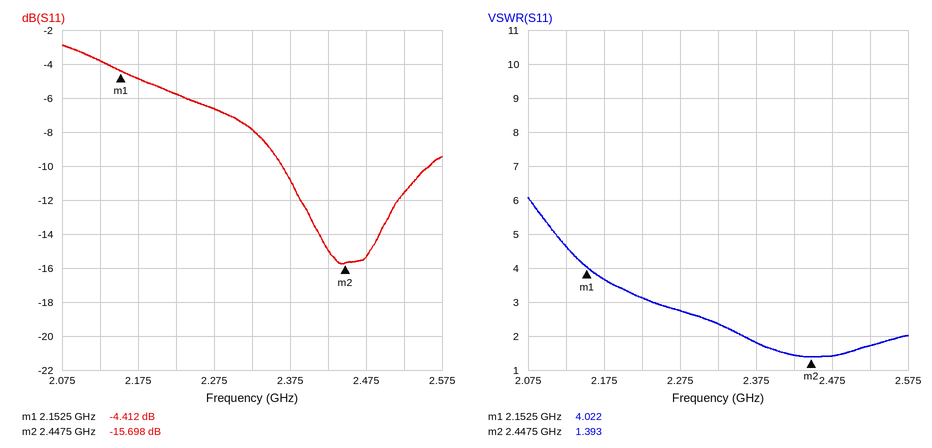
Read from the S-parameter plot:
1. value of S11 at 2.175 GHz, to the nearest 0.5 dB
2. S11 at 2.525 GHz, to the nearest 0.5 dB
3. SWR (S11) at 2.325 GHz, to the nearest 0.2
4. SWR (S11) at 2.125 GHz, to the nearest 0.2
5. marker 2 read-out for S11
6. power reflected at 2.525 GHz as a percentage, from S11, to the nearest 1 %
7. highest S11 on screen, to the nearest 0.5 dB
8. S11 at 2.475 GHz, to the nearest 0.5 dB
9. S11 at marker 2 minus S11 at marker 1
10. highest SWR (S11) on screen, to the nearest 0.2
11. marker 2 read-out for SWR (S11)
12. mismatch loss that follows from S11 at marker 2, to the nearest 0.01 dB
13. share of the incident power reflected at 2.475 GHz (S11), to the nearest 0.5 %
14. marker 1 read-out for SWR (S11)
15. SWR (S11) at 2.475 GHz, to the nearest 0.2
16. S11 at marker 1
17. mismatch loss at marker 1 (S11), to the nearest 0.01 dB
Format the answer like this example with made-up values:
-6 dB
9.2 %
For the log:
-5.0 dB
-11.5 dB
2.4
4.6
-15.698 dB
7 %
-3.0 dB
-15.5 dB
-11.286 dB
6.0
1.393
0.12 dB
3.0 %
4.022
1.4
-4.412 dB
1.95 dB
